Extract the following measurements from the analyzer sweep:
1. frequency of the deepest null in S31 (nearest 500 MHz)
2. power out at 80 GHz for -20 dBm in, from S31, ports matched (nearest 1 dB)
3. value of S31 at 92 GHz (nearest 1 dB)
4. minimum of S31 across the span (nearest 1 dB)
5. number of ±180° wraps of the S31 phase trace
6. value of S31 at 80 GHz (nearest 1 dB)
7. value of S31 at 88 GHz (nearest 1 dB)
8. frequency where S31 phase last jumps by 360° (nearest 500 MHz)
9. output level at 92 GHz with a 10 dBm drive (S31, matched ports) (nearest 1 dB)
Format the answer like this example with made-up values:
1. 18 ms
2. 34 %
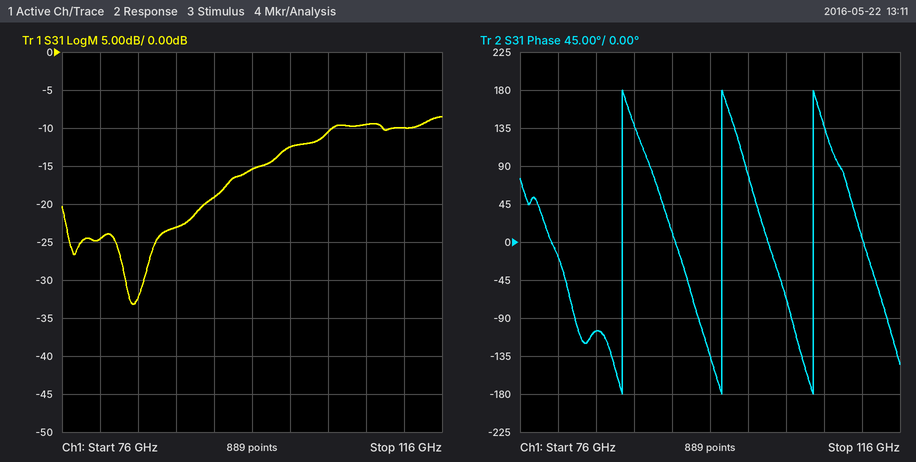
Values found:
1. 83.5 GHz
2. -45 dBm
3. -19 dB
4. -33 dB
5. 3
6. -25 dB
7. -23 dB
8. 107.0 GHz
9. -9 dBm
